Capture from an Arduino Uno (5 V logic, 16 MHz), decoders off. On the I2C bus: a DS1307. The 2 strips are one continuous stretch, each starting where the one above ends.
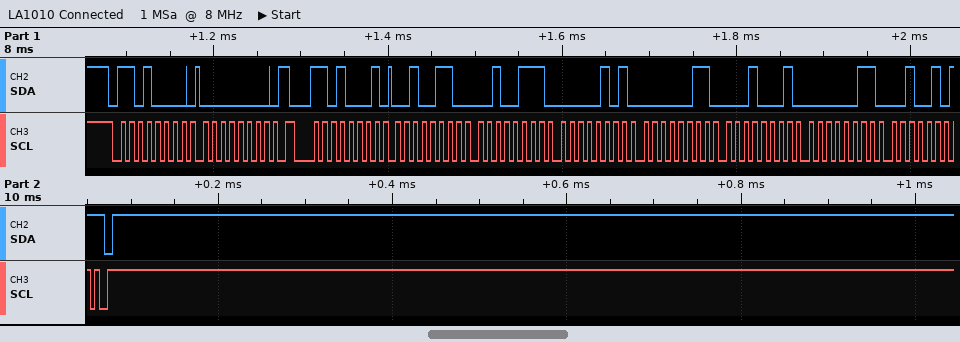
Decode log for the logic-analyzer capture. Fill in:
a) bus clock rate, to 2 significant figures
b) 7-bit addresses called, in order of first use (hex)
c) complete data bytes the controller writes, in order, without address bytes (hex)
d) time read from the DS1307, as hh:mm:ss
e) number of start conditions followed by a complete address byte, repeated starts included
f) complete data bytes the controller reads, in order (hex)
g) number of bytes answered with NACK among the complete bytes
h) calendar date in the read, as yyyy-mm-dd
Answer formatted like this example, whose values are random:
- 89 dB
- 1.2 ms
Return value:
- 100 kHz
- 0x68
- 00
- 05:27:26
- 2
- 26 27 05 03 11 03 25
- 1
- 2025-03-11
